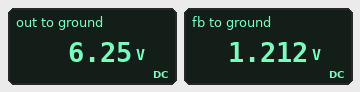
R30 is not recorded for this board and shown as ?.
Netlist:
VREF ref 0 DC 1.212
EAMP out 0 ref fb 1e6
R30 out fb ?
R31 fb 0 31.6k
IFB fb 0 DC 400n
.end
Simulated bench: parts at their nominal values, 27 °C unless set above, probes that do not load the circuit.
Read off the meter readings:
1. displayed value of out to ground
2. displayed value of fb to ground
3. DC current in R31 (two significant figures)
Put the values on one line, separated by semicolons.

6.25 V; 1.212 V; 38 µA
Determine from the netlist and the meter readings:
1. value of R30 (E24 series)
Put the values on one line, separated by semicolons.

130 kΩ
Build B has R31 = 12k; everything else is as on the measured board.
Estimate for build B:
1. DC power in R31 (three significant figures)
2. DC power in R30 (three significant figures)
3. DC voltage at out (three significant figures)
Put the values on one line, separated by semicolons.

122 µW; 1.34 mW; 14.4 V
